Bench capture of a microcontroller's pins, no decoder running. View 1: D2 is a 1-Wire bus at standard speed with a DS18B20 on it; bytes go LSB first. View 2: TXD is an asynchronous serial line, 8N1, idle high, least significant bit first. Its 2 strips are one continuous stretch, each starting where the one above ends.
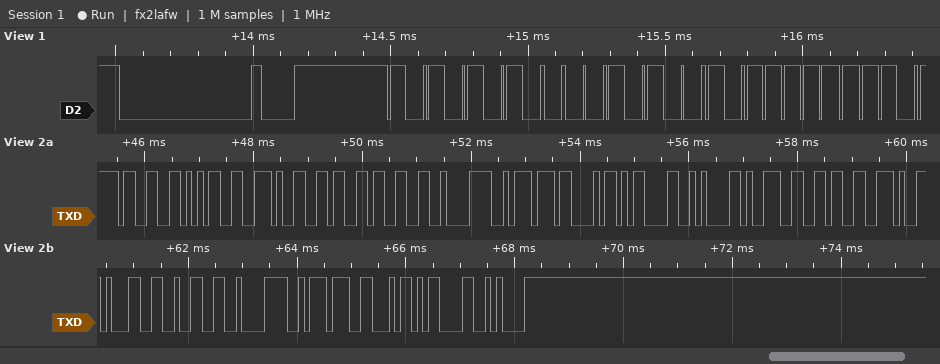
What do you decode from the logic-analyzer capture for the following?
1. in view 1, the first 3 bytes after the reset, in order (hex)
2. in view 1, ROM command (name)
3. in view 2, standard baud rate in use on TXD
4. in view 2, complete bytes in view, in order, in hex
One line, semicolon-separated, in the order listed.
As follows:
55 28 FD; Match ROM; 9600 baud; 0x33 0x35 0x2E 0x36 0x33 0xC2 0xBA 0x43 0x0D 0x0A 0x39 0x36 0x2E 0x31 0x32 0xC2 0xBA 0x46 0x0D 0x0A
